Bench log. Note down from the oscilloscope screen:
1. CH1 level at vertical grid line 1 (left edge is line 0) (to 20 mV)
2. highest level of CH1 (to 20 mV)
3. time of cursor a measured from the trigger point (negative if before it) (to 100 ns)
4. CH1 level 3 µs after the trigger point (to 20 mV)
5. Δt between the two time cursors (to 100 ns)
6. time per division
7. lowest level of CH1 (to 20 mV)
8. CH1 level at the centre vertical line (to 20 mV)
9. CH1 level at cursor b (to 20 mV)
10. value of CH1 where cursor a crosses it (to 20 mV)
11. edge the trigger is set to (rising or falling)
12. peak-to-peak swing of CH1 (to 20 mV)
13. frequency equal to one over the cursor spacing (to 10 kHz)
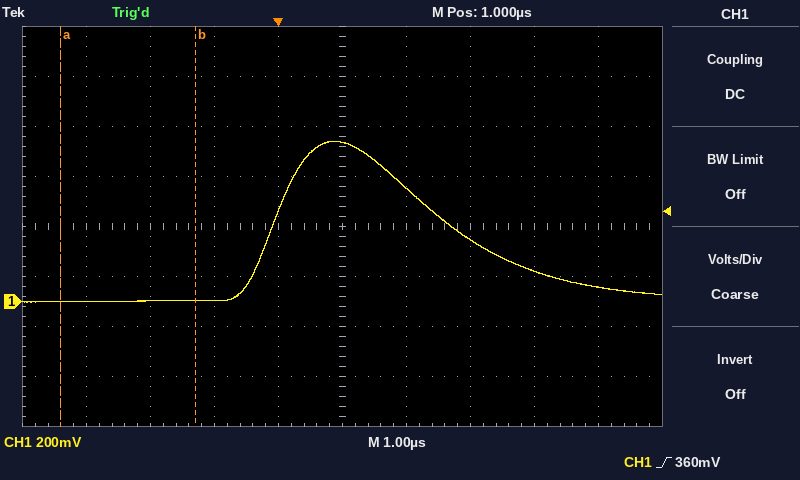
0 mV
640 mV
-3.4 µs
240 mV
2.1 µs
1 µs
0 mV
640 mV
0 mV
0 mV
rising
640 mV
480 kHz
